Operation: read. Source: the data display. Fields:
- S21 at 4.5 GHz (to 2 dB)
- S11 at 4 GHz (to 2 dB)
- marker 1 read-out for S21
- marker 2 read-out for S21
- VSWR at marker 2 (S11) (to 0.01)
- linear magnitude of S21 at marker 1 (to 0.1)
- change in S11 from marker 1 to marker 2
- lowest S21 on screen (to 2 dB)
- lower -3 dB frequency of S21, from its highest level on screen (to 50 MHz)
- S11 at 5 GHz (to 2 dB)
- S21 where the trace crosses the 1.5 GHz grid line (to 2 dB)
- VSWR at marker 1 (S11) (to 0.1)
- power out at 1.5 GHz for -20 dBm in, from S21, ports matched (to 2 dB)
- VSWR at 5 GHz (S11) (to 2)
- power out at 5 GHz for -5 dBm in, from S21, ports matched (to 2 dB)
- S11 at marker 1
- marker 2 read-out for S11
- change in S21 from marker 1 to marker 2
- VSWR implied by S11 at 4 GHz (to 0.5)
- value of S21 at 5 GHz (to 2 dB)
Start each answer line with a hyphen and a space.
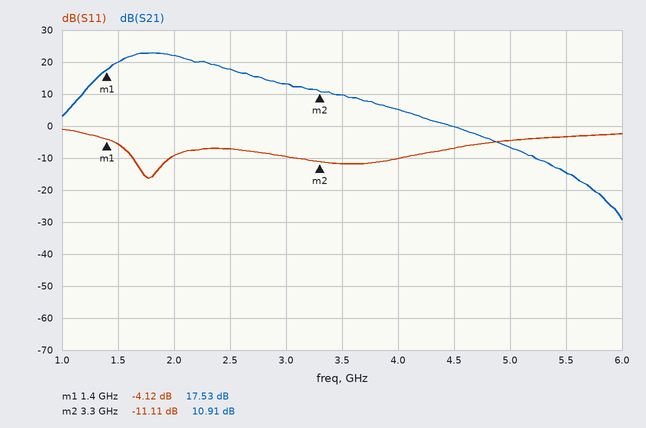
- 0 dB
- -10 dB
- 17.53 dB
- 10.91 dB
- 1.77
- 7.5
- -6.99 dB
- -30 dB
- 1.50 GHz
- -4 dB
- 20 dB
- 4.3
- 0 dBm
- 4
- -12 dBm
- -4.12 dB
- -11.11 dB
- -6.62 dB
- 2.0
- -6 dB
